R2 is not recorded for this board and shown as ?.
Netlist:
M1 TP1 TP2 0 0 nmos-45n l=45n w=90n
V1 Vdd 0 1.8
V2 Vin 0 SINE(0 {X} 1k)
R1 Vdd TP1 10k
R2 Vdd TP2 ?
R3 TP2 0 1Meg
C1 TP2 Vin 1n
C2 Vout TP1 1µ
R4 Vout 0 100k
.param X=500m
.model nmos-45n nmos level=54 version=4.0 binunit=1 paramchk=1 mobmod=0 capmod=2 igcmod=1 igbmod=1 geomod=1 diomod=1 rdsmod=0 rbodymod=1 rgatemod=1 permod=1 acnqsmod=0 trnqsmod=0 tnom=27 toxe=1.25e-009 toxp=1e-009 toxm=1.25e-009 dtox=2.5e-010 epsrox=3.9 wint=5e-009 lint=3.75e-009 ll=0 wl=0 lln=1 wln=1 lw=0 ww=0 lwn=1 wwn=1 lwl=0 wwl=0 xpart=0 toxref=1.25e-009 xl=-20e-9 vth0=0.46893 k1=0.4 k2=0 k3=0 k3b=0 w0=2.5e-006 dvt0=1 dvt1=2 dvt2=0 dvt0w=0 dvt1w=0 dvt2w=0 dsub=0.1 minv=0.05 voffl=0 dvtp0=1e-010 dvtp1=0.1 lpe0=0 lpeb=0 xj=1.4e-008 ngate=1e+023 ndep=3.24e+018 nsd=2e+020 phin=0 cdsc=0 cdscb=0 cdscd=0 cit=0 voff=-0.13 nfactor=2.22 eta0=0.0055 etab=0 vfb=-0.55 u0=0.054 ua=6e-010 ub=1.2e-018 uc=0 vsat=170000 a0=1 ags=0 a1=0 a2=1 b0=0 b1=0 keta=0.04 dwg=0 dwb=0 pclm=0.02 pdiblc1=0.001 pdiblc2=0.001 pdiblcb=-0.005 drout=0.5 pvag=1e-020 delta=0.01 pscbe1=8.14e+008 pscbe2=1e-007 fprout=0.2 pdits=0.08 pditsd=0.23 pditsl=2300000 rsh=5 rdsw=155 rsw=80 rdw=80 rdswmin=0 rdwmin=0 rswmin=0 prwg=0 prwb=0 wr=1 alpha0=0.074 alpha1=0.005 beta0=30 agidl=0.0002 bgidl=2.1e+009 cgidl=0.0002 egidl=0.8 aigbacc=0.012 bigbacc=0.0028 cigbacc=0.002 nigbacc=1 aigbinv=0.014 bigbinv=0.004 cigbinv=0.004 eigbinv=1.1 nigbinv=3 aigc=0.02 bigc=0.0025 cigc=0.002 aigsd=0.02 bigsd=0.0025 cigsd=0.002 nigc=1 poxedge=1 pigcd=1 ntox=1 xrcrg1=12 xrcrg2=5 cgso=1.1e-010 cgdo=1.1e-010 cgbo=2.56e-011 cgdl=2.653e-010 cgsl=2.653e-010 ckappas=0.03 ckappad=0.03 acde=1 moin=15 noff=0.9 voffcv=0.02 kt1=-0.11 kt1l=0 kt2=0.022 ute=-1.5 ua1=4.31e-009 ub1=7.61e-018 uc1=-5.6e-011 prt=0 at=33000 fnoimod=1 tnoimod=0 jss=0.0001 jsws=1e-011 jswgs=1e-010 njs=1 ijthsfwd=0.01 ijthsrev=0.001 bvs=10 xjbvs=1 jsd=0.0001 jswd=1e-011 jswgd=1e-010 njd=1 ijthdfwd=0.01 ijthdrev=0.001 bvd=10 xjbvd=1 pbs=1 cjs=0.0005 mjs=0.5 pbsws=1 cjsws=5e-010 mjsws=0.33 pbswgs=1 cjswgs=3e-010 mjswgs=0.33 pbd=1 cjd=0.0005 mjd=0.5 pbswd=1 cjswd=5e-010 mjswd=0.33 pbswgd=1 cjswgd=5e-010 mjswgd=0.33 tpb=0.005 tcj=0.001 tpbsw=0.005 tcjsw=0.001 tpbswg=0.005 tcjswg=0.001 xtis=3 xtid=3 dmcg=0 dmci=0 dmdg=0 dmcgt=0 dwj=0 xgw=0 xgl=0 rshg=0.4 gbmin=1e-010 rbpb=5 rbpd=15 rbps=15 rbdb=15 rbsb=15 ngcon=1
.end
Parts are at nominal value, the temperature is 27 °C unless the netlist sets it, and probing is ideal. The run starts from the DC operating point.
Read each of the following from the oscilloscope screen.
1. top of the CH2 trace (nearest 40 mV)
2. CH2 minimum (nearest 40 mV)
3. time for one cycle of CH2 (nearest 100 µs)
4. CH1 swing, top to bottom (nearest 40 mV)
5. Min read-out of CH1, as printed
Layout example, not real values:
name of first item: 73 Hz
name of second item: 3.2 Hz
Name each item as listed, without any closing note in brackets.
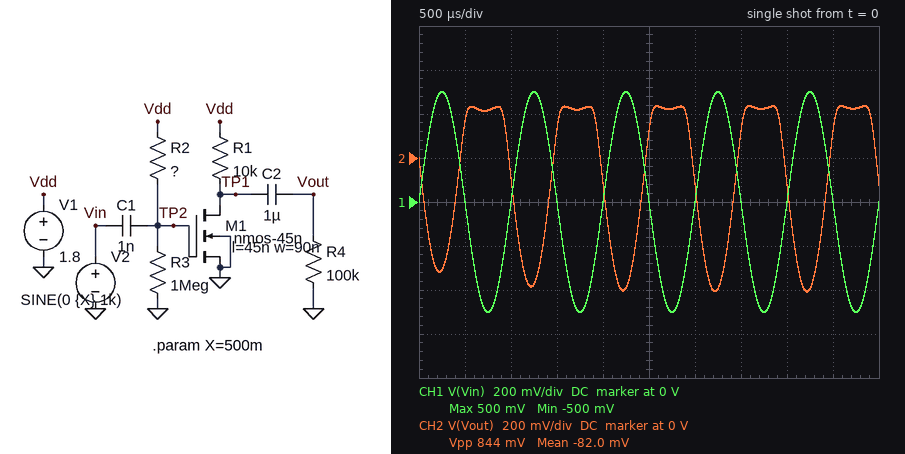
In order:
top of the CH2 trace: 240 mV
CH2 minimum: -600 mV
time for one cycle of CH2: 1.0 ms
CH1 swing, top to bottom: 1.00 V
Min read-out of CH1, as printed: -500 mV
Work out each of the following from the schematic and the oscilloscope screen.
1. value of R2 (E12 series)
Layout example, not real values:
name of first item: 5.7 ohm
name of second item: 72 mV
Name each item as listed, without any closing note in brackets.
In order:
value of R2: 3.3 MΩ
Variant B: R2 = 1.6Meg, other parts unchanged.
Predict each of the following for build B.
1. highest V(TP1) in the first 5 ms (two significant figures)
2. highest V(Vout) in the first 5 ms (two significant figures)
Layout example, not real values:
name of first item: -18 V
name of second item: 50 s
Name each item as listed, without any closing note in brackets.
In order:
highest V(TP1) in the first 5 ms: 1.7 V
highest V(Vout) in the first 5 ms: 560 mV
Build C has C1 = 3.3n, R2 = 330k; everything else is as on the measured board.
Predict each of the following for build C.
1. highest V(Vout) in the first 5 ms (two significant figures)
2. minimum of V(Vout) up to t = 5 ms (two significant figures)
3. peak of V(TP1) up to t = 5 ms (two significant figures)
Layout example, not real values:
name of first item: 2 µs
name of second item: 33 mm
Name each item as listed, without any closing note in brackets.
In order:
highest V(Vout) in the first 5 ms: 500 mV
minimum of V(Vout) up to t = 5 ms: -69 mV
peak of V(TP1) up to t = 5 ms: 960 mV
